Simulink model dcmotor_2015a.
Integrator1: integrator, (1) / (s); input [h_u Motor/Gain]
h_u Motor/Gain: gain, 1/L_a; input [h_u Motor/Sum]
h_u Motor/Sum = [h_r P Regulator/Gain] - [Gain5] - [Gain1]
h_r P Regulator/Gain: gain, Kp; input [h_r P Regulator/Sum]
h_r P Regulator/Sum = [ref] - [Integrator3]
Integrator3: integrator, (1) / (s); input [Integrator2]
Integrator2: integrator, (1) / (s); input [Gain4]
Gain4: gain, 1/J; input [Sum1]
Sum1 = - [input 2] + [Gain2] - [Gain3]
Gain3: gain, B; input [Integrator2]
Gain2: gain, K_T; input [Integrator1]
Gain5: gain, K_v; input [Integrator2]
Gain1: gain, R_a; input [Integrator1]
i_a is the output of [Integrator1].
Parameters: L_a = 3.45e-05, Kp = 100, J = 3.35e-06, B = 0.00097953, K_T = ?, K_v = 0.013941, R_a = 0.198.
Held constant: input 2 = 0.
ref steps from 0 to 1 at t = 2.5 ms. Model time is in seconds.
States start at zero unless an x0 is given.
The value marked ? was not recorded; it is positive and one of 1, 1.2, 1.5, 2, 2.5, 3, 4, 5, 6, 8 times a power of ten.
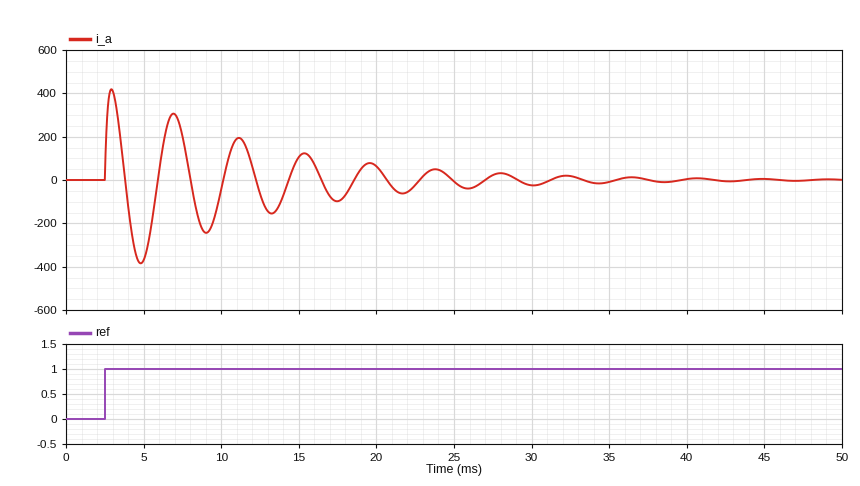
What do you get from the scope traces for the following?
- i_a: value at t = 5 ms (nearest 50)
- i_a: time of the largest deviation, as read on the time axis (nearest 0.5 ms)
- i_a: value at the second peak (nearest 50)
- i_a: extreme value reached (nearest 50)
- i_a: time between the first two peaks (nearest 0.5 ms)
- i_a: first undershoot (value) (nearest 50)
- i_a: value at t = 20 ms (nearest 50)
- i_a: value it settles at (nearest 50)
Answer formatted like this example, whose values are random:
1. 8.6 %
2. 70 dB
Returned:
1. -350
2. 3.0 ms
3. 300
4. 400
5. 4.0 ms
6. -400
7. 50
8. 0
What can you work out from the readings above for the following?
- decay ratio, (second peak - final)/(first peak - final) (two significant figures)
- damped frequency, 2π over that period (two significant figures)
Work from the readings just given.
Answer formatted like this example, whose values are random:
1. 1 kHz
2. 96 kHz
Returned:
1. 0.75
2. 1.6 rad/ms
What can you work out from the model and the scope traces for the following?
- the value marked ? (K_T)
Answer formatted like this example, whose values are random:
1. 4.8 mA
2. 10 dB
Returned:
1. 0.015
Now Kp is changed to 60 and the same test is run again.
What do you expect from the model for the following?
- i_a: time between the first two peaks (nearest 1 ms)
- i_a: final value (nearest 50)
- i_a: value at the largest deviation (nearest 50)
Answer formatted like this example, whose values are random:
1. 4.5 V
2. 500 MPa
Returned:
1. 5 ms
2. 0
3. 250
